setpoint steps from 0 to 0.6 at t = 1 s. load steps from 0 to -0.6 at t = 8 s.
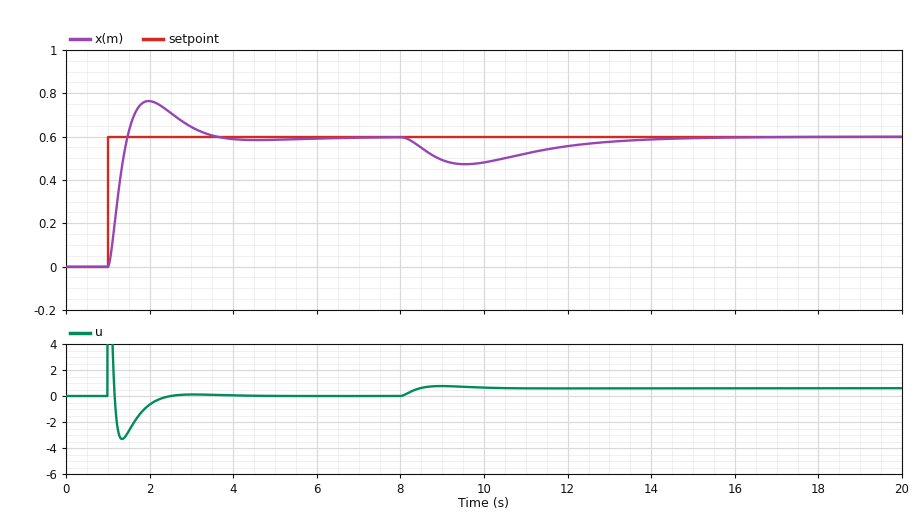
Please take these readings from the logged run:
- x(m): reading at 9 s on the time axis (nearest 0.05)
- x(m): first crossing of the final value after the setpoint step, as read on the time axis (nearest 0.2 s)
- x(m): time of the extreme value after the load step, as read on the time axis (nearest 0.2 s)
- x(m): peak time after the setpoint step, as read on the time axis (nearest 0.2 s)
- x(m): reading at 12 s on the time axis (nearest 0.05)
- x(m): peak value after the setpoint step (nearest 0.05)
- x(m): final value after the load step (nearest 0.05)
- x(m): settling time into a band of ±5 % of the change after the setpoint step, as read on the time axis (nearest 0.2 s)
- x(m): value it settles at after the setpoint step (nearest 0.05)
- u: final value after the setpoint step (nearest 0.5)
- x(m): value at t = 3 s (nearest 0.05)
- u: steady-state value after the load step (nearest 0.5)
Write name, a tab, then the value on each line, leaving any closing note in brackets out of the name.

x(m): reading at 9 s on the time axis	0.50
x(m): first crossing of the final value after the setpoint step, as read on the time axis	1.4 s
x(m): time of the extreme value after the load step, as read on the time axis	9.6 s
x(m): peak time after the setpoint step, as read on the time axis	2.0 s
x(m): reading at 12 s on the time axis	0.55
x(m): peak value after the setpoint step	0.75
x(m): final value after the load step	0.60
x(m): settling time into a band of ±5 % of the change after the setpoint step, as read on the time axis	3.2 s
x(m): value it settles at after the setpoint step	0.60
u: final value after the setpoint step	0.0
x(m): value at t = 3 s	0.65
u: steady-state value after the load step	0.5
